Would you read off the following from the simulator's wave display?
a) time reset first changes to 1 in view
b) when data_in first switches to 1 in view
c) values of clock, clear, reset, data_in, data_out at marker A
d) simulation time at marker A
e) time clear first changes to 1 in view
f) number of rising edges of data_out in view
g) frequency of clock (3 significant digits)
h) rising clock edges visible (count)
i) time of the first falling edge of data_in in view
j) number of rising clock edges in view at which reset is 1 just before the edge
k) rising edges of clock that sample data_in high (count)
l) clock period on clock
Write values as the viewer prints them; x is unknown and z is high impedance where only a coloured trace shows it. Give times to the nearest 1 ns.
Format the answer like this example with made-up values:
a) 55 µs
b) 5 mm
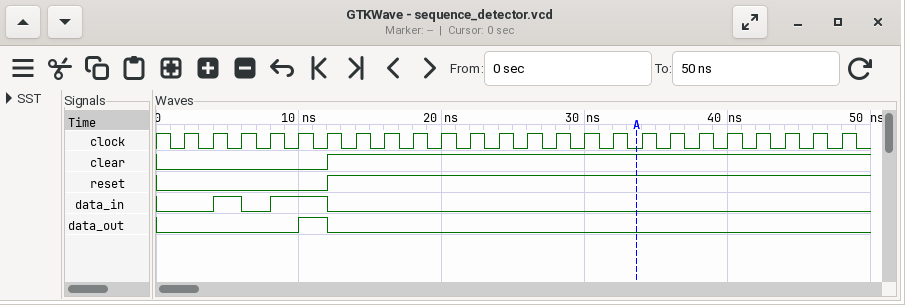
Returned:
a) 12 ns
b) 4 ns
c) clock=0, clear=1, reset=1, data_in=0, data_out=0
d) 34 ns
e) 12 ns
f) 1
g) 500 MHz
h) 24
i) 6 ns
j) 18
k) 3
l) 2 ns
